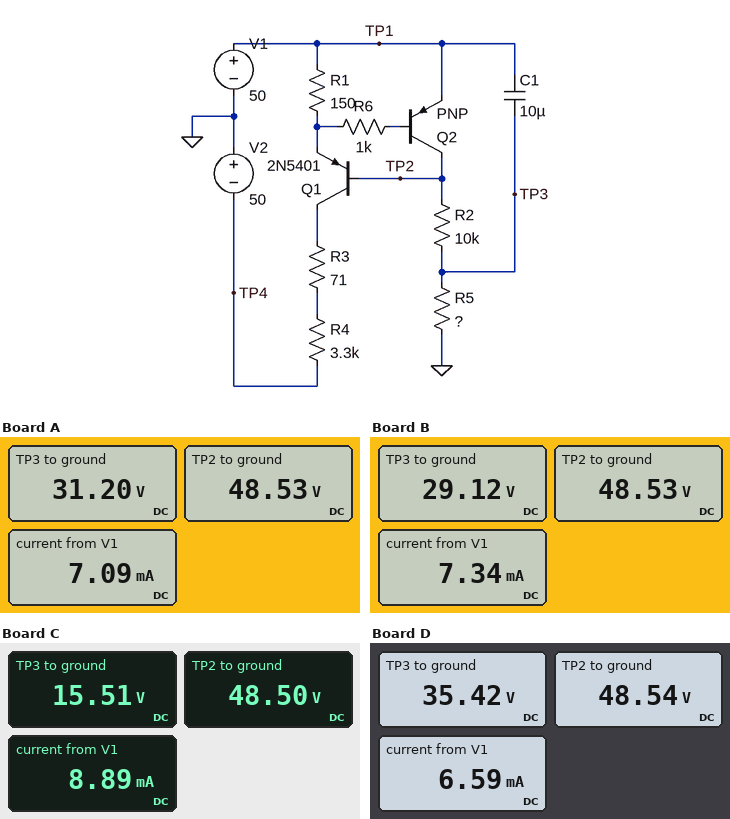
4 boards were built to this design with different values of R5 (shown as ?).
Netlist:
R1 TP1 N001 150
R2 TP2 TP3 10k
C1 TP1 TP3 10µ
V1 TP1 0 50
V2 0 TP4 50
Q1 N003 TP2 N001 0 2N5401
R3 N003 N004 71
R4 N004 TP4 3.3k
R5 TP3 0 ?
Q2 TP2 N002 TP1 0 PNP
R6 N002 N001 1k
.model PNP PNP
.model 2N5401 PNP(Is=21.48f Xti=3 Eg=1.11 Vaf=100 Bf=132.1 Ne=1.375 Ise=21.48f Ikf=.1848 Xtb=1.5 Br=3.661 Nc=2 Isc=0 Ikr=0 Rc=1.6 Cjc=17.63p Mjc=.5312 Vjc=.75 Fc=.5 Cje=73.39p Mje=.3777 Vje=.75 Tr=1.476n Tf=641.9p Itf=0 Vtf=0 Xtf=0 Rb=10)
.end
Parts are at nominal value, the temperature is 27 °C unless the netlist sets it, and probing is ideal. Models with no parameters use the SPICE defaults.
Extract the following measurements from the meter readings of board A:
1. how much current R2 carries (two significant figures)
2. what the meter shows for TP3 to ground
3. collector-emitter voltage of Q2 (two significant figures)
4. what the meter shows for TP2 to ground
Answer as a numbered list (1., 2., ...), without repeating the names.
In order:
1. 1.7 mA
2. 31.20 V
3. -1.5 V
4. 48.53 V
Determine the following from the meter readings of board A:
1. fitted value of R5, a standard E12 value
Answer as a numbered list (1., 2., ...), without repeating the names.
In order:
1. 18 kΩ
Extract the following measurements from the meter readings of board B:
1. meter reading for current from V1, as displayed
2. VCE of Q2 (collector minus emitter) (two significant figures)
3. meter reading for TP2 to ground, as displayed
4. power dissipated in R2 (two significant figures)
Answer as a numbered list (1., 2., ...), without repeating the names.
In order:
1. 7.34 mA
2. -1.5 V
3. 48.53 V
4. 38 mW
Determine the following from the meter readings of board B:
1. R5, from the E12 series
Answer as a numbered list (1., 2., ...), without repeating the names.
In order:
1. 15 kΩ
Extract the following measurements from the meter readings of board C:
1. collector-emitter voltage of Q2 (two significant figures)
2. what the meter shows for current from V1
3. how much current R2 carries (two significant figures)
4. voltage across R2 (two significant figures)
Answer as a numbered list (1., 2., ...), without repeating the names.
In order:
1. -1.5 V
2. 8.89 mA
3. 3.3 mA
4. 33 V
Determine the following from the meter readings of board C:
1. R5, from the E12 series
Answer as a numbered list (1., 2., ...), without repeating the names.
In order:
1. 4.7 kΩ
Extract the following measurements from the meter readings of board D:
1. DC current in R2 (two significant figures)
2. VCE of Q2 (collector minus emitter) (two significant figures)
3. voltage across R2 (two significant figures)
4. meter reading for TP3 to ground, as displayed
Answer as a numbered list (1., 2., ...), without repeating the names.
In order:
1. 1.3 mA
2. -1.5 V
3. 13 V
4. 35.42 V
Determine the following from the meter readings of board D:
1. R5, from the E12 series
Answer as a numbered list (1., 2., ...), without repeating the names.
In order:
1. 27 kΩ
